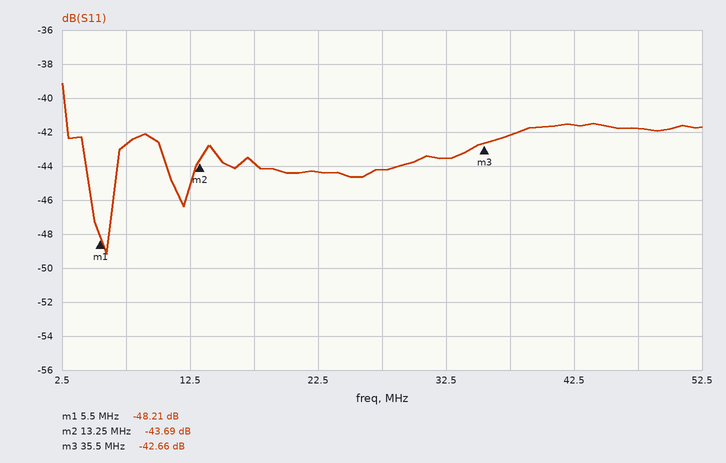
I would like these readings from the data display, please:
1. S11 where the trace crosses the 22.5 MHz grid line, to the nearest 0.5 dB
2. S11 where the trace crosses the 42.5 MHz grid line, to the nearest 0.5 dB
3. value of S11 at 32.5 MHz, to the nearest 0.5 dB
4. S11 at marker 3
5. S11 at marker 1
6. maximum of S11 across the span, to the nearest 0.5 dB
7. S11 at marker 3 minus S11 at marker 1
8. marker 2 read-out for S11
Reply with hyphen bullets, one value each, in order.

- -44.5 dB
- -41.5 dB
- -43.5 dB
- -42.66 dB
- -48.21 dB
- -39.0 dB
- 5.55 dB
- -43.69 dB
